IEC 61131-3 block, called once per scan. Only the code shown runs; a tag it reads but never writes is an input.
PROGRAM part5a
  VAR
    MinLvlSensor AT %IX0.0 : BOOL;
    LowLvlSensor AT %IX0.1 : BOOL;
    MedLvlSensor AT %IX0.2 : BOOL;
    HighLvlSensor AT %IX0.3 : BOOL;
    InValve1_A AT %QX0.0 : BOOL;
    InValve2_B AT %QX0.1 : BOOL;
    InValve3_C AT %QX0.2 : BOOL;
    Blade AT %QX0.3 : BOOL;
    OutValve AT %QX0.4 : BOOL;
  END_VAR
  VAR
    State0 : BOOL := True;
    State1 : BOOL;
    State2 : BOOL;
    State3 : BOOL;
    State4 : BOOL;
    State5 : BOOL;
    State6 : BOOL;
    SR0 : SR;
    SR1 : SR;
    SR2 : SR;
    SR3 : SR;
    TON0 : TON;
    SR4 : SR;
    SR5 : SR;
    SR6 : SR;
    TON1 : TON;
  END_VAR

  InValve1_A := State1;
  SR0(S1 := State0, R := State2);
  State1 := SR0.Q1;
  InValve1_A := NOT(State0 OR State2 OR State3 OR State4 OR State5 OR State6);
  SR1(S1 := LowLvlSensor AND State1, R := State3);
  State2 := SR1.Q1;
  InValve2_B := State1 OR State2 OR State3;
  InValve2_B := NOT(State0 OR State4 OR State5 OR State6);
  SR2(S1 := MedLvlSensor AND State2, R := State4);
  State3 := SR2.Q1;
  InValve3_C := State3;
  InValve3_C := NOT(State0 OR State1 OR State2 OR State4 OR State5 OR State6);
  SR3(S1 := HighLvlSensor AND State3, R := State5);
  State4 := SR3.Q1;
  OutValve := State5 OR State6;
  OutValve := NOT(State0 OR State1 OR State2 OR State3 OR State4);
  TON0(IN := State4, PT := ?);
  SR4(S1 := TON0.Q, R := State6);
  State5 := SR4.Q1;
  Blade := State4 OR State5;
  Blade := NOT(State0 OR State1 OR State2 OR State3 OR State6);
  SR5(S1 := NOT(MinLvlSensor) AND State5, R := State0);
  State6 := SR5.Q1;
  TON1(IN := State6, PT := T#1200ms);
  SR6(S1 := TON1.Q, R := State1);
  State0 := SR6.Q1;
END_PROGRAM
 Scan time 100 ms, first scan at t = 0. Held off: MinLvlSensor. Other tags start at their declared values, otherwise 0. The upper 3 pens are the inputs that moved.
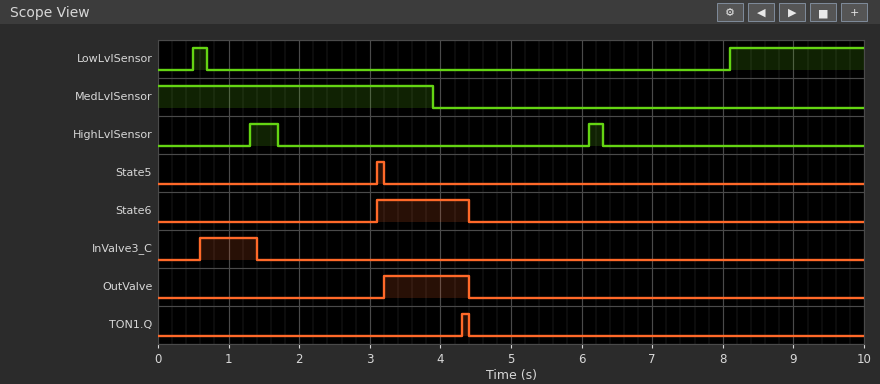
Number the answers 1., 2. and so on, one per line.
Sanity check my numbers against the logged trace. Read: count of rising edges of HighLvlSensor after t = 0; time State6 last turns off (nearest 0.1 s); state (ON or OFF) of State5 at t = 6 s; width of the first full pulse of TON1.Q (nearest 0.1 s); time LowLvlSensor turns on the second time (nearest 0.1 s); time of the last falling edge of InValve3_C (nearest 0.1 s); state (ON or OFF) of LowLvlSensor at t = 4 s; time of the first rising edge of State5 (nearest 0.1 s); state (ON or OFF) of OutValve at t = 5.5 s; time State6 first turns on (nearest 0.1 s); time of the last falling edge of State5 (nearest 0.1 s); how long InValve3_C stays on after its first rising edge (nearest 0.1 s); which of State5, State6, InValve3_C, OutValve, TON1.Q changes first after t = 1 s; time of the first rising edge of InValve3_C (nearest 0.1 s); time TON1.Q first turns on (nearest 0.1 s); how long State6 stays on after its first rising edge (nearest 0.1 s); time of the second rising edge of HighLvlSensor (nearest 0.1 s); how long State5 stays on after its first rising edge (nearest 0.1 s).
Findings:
1. 2
2. 4.4 s
3. OFF
4. 0.1 s
5. 8.1 s
6. 1.4 s
7. OFF
8. 3.1 s
9. OFF
10. 3.1 s
11. 3.2 s
12. 0.8 s
13. InValve3_C
14. 0.6 s
15. 4.3 s
16. 1.3 s
17. 6.1 s
18. 0.1 s
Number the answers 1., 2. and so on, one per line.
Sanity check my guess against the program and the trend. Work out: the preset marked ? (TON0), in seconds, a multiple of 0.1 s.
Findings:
1. 1.8 s
